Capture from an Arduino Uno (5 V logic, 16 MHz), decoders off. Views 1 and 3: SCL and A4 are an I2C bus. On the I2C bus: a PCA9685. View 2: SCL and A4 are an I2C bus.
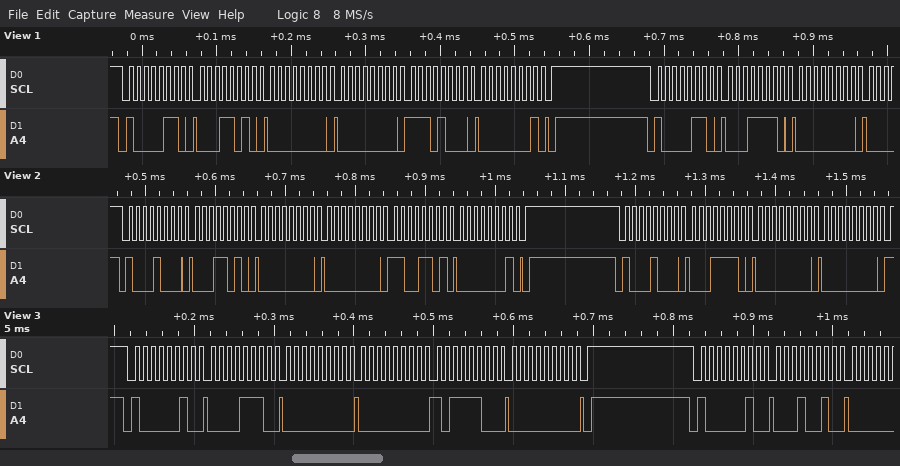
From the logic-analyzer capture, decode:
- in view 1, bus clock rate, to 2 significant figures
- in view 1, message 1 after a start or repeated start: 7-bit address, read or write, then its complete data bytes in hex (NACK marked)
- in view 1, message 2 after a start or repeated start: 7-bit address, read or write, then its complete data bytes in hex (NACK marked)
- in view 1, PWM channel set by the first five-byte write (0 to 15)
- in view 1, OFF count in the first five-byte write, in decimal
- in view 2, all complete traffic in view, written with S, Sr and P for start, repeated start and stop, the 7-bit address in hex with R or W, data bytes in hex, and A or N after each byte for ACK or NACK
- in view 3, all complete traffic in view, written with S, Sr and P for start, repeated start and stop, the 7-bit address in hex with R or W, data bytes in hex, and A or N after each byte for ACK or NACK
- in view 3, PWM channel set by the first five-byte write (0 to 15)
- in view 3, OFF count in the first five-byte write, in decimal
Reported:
100 kHz
0x43 write: 1A 00 00 E8 01
0x43 write: 1E 00
5
488
S 44W A 1A A 00 A 00 A CD A 01 A P S 44W A 1E A 00 A 00 A
S 41W A 0E A 00 A 00 A BC A 00 A P S 41W A 12 A
2
188
